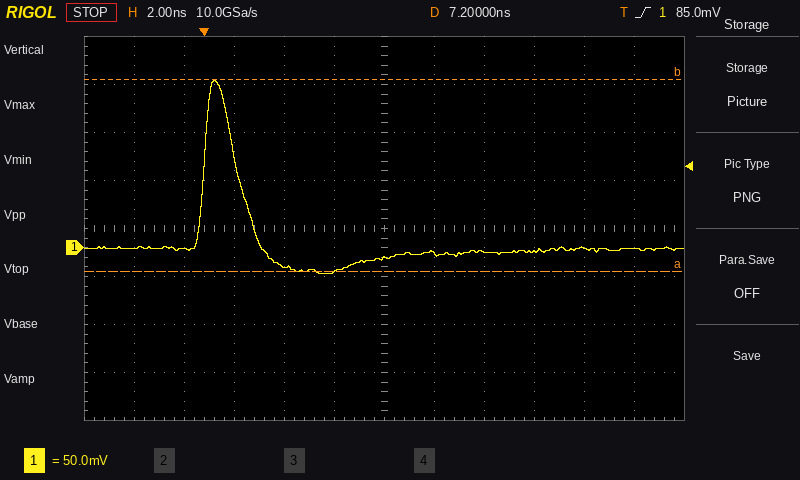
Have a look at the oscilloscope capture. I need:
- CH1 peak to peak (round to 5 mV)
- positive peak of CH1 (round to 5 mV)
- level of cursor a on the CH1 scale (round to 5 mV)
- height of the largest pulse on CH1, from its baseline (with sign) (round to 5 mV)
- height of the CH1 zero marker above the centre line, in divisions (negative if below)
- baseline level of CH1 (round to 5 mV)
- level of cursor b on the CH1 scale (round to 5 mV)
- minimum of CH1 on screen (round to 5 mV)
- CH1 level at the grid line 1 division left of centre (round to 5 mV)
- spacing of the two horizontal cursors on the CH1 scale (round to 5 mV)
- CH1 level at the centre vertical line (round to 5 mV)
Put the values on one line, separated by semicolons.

200 mV; 175 mV; -25 mV; +175 mV; -0.4 div; 0 mV; 175 mV; -25 mV; -25 mV; 200 mV; -10 mV
